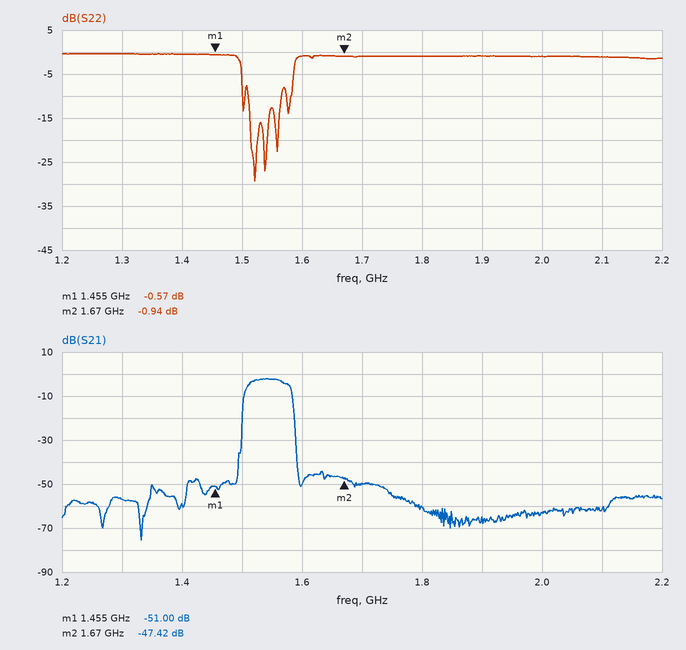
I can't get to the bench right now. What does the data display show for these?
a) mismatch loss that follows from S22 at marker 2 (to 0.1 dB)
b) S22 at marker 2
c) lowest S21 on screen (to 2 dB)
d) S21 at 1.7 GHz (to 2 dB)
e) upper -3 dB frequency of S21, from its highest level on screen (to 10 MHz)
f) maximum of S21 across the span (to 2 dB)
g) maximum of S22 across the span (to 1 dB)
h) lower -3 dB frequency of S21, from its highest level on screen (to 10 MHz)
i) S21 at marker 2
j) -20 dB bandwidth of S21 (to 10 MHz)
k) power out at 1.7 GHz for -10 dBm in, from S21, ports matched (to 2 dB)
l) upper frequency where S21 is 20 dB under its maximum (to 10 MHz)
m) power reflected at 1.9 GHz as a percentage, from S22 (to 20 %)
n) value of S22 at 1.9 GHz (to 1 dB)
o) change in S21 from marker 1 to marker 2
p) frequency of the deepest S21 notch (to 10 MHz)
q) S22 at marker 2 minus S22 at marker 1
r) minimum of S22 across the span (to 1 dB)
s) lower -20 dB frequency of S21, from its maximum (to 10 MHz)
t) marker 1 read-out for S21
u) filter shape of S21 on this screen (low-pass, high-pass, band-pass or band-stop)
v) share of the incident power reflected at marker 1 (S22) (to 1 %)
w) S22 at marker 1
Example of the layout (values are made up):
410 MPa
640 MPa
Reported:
7.1 dB
-0.94 dB
-76 dB
-50 dB
1.58 GHz
-2 dB
0 dB
1.51 GHz
-47.42 dB
90 MHz
-60 dBm
1.59 GHz
80 %
-1 dB
3.58 dB
1.33 GHz
-0.37 dB
-29 dB
1.50 GHz
-51.00 dB
band-pass
88 %
-0.57 dB
